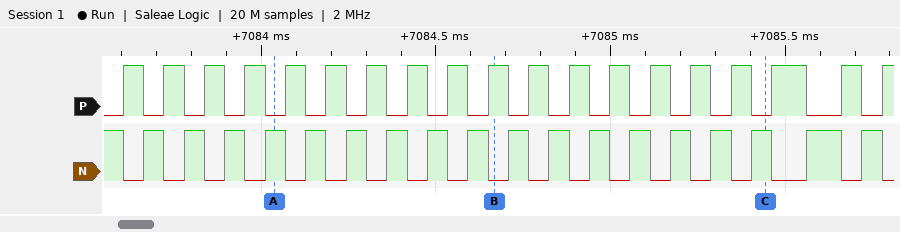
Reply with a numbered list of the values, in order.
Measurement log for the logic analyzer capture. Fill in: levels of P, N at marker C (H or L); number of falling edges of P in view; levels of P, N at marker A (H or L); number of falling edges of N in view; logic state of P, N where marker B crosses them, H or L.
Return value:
1. P=L, N=H
2. 18
3. P=L, N=H
4. 19
5. P=H, N=L
